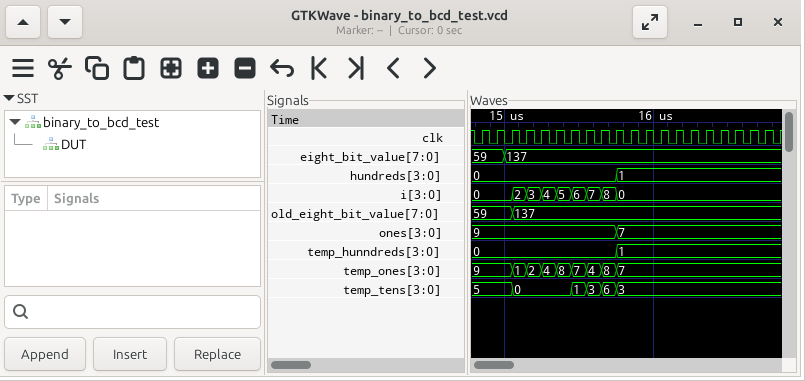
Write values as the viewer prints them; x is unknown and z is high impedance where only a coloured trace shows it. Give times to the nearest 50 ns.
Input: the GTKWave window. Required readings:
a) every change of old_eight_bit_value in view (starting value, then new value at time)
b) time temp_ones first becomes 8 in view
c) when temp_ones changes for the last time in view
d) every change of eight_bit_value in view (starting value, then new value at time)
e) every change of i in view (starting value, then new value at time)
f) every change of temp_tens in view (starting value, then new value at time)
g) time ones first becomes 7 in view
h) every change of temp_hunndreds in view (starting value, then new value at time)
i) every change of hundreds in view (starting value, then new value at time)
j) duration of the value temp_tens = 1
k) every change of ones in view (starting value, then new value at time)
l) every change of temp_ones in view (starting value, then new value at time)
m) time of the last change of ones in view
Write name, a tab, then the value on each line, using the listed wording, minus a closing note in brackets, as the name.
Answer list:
every change of old_eight_bit_value in view	59, 137 at 15050 ns
time temp_ones first becomes 8 in view	15350 ns
when temp_ones changes for the last time in view	15750 ns
every change of eight_bit_value in view	59, 137 at 15000 ns
every change of i in view	0, 2 at 15050 ns, 3 at 15150 ns, 4 at 15250 ns, 5 at 15350 ns, 6 at 15450 ns, 7 at 15550 ns, 8 at 15650 ns, 0 at 15750 ns
every change of temp_tens in view	5, 0 at 15050 ns, 1 at 15450 ns, 3 at 15550 ns, 6 at 15650 ns, 3 at 15750 ns
time ones first becomes 7 in view	15750 ns
every change of temp_hunndreds in view	0, 1 at 15750 ns
every change of hundreds in view	0, 1 at 15750 ns
duration of the value temp_tens = 1	100 ns
every change of ones in view	9, 7 at 15750 ns
every change of temp_ones in view	9, 1 at 15050 ns, 2 at 15150 ns, 4 at 15250 ns, 8 at 15350 ns, 7 at 15450 ns, 4 at 15550 ns, 8 at 15650 ns, 7 at 15750 ns
time of the last change of ones in view	15750 ns
